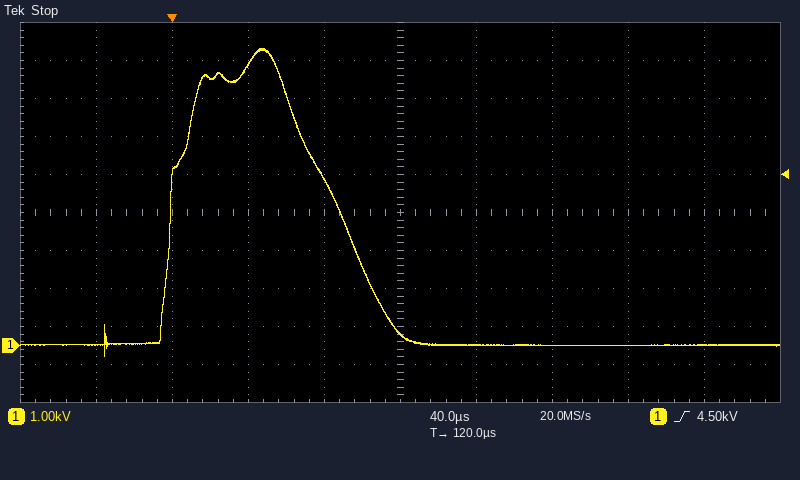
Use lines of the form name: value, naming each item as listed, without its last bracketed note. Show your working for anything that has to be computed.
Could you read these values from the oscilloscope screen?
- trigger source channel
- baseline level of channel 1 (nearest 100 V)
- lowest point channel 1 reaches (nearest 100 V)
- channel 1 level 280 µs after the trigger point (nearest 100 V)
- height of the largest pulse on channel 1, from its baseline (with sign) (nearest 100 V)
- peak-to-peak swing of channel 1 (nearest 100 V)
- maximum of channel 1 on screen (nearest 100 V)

trigger source channel: channel 1
baseline level of channel 1: 0.0 kV
lowest point channel 1 reaches: -300 V
channel 1 level 280 µs after the trigger point: 0.0 kV
height of the largest pulse on channel 1, from its baseline (with sign): 7.8 kV − (0.0 kV) = +7.8 kV
peak-to-peak swing of channel 1: 7.8 kV − (-300 V) = 8.1 kV
maximum of channel 1 on screen: 7.8 kV
